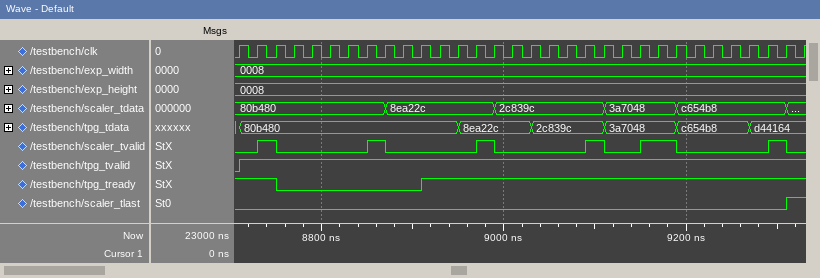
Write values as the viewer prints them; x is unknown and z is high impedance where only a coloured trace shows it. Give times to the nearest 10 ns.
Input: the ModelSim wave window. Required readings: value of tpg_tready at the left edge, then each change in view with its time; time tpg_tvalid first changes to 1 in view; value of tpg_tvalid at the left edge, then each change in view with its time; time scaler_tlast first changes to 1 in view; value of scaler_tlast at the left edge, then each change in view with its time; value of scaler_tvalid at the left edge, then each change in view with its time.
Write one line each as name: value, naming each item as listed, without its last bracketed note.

value of tpg_tready at the left edge, then each change in view with its time: 1, 0 at 8750 ns, 1 at 8910 ns
time tpg_tvalid first changes to 1 in view: 8710 ns
value of tpg_tvalid at the left edge, then each change in view with its time: 0, 1 at 8710 ns
time scaler_tlast first changes to 1 in view: 9310 ns
value of scaler_tlast at the left edge, then each change in view with its time: 0, 1 at 9310 ns
value of scaler_tvalid at the left edge, then each change in view with its time: 0, 1 at 8730 ns, 0 at 8750 ns, 1 at 8850 ns, 0 at 8870 ns, 1 at 8970 ns, 0 at 8990 ns, 1 at 9090 ns, 0 at 9110 ns, 1 at 9150 ns, 0 at 9190 ns, 1 at 9290 ns, 0 at 9310 ns
